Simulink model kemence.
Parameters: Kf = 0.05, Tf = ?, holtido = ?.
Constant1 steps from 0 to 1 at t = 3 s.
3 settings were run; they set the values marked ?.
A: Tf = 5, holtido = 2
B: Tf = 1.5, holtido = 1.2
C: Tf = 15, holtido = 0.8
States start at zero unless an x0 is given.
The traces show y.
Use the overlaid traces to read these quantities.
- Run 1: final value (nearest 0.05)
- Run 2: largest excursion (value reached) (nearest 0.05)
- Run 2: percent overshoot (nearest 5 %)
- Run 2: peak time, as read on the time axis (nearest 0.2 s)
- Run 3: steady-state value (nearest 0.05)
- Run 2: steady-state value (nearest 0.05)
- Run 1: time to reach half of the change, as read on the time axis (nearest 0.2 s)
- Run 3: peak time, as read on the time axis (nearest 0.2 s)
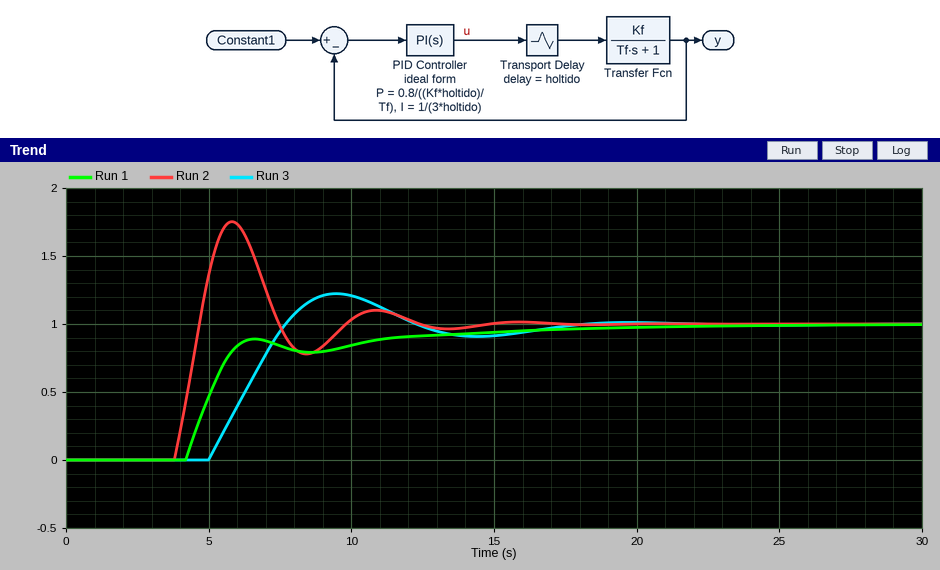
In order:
1.00
1.75
75 %
5.8 s
1.00
1.00
5.0 s
9.4 s
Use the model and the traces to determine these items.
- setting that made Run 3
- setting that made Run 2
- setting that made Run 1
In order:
A
C
B
